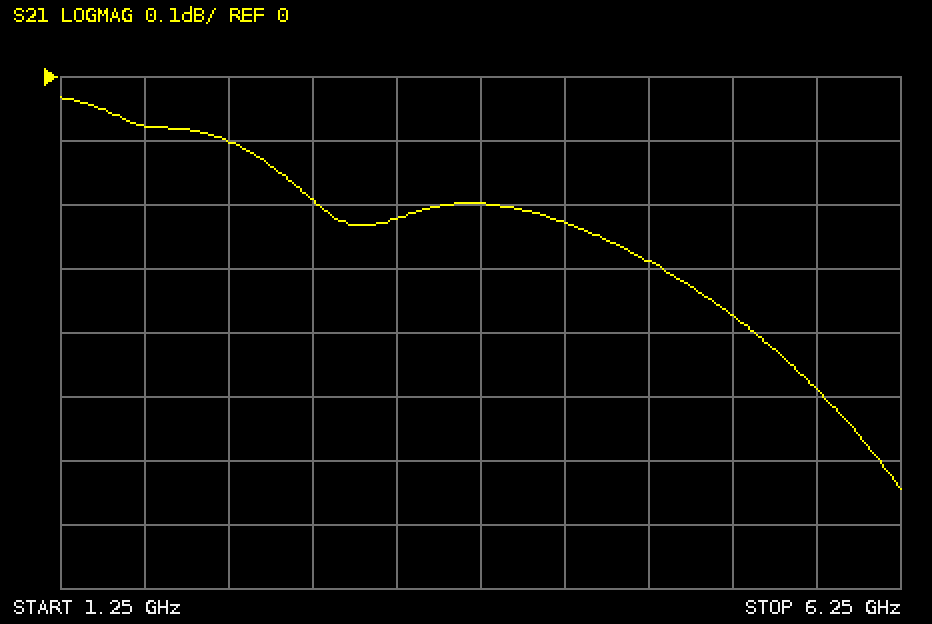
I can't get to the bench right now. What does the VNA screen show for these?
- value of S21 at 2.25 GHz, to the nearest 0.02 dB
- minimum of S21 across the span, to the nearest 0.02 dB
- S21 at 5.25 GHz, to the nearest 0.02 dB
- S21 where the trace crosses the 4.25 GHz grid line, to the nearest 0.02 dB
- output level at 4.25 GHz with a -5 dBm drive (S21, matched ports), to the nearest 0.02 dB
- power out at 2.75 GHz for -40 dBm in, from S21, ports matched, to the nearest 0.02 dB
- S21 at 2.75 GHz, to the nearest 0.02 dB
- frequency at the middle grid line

-0.10 dB
-0.64 dB
-0.38 dB
-0.22 dB
-5.22 dBm
-40.20 dBm
-0.20 dB
3.75 GHz
